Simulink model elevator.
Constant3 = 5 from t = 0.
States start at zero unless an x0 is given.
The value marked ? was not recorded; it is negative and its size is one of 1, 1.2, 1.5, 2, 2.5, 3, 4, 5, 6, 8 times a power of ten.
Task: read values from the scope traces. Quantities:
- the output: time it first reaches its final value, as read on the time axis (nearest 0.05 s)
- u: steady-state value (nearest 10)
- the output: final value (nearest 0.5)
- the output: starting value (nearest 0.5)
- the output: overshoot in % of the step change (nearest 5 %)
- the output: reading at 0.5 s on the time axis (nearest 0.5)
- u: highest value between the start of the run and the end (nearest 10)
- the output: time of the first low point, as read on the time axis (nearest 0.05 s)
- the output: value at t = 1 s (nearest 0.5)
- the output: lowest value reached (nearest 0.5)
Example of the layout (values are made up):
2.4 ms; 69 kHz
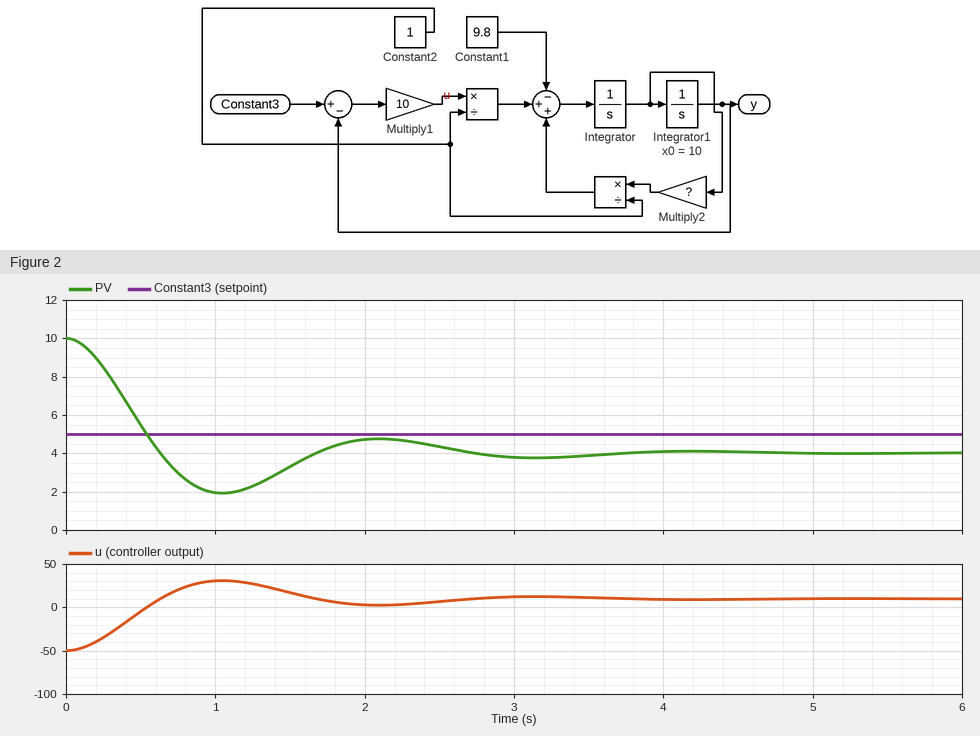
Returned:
0.65 s; 10; 4.0; 10.0; 35 %; 5.5; 30; 1.05 s; 2.0; 2.0
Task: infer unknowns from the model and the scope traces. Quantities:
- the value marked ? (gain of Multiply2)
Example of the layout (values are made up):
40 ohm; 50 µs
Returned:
-2
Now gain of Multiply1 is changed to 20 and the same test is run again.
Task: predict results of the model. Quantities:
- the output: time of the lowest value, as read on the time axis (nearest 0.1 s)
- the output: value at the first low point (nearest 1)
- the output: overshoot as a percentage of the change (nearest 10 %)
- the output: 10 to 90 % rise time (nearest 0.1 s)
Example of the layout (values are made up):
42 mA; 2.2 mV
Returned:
0.7 s; 2; 50 %; 0.3 s
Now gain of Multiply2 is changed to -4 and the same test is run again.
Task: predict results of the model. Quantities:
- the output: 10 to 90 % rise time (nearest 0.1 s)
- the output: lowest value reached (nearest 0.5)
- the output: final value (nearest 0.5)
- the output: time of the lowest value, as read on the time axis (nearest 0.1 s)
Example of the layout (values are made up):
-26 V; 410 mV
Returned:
0.6 s; 3.5; 4.0; 1.3 s
